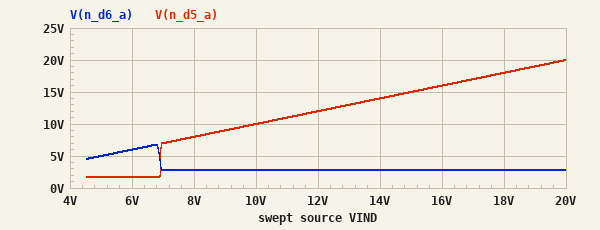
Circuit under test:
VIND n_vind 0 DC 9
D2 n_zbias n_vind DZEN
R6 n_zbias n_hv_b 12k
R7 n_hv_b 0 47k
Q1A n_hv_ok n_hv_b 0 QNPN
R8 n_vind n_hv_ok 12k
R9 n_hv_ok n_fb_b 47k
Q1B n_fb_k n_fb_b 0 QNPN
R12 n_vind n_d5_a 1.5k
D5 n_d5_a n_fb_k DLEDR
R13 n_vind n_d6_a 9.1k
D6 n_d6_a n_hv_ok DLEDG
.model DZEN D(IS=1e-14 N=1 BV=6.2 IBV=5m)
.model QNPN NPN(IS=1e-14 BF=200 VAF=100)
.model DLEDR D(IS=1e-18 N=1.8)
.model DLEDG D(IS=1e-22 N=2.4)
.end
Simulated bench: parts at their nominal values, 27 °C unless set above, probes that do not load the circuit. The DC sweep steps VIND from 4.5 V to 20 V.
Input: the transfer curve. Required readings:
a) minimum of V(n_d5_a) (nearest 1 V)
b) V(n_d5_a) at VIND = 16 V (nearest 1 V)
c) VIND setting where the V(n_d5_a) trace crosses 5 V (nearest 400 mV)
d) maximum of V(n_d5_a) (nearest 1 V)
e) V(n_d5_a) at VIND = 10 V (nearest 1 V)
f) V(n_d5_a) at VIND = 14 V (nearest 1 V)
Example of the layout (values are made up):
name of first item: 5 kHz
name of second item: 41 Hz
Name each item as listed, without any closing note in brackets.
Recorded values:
minimum of V(n_d5_a): 2 V
V(n_d5_a) at VIND = 16 V: 16 V
VIND setting where the V(n_d5_a) trace crosses 5 V: 6.8 V
maximum of V(n_d5_a): 20 V
V(n_d5_a) at VIND = 10 V: 10 V
V(n_d5_a) at VIND = 14 V: 14 V
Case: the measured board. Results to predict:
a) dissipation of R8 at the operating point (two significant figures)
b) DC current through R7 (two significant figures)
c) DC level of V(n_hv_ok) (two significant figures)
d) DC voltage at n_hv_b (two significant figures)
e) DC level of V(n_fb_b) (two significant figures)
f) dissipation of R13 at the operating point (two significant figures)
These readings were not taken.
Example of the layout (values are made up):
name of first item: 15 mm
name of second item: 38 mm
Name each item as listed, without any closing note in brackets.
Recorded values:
dissipation of R8 at the operating point: 6.7 mW
DC current through R7: 14 µA
DC level of V(n_hv_ok): 62 mV
DC voltage at n_hv_b: 670 mV
DC level of V(n_fb_b): 62 mV
dissipation of R13 at the operating point: 4.3 mW
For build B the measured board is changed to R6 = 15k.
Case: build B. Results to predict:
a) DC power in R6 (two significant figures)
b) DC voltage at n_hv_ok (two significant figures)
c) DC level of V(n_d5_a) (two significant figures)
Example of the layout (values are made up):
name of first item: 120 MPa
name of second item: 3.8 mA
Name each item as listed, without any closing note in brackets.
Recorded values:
DC power in R6: 330 µW
DC voltage at n_hv_ok: 67 mV
DC level of V(n_d5_a): 9.0 V
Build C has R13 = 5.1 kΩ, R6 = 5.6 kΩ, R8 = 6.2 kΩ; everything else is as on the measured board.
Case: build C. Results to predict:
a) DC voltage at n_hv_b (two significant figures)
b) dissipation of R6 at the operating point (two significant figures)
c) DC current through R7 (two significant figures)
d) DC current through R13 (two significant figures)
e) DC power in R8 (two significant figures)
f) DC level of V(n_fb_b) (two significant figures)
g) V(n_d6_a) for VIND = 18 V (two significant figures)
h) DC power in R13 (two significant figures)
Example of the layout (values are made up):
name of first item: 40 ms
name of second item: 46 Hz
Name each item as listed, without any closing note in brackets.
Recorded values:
DC voltage at n_hv_b: 690 mV
dissipation of R6 at the operating point: 850 µW
DC current through R7: 15 µA
DC current through R13: 1.2 mA
DC power in R8: 13 mW
DC level of V(n_fb_b): 58 mV
V(n_d6_a) for VIND = 18 V: 2.8 V
DC power in R13: 7.6 mW
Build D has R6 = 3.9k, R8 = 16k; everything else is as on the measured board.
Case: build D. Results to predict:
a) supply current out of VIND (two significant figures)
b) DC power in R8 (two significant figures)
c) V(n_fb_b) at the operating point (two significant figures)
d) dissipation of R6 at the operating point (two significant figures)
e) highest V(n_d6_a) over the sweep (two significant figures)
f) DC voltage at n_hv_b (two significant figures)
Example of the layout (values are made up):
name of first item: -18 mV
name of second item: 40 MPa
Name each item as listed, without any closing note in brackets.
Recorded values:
supply current out of VIND: 1.8 mA
DC power in R8: 5.0 mW
V(n_fb_b) at the operating point: 38 mV
dissipation of R6 at the operating point: 1.2 mW
highest V(n_d6_a) over the sweep: 6.7 V
DC voltage at n_hv_b: 680 mV
